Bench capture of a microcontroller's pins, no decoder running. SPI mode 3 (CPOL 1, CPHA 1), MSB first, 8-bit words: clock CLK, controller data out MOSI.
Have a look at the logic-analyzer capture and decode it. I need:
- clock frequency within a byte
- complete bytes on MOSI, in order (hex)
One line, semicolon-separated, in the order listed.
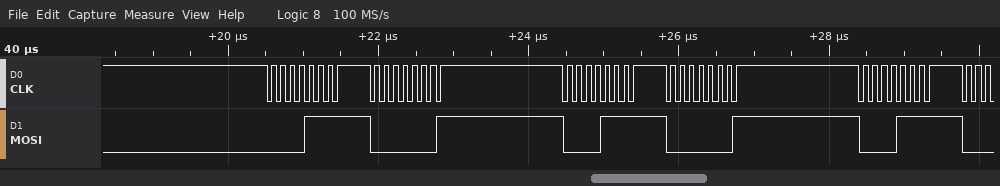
8 MHz; 0F 01 0F 01 0F
